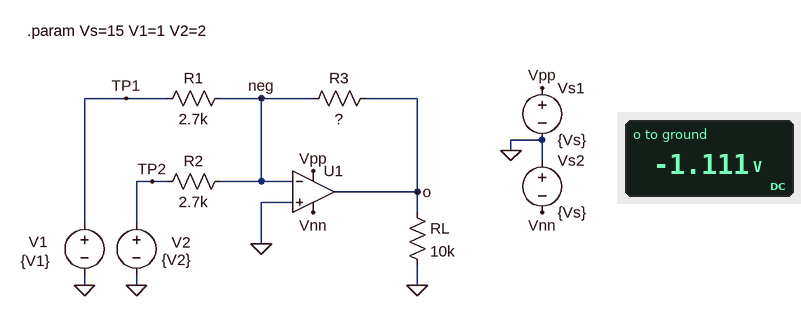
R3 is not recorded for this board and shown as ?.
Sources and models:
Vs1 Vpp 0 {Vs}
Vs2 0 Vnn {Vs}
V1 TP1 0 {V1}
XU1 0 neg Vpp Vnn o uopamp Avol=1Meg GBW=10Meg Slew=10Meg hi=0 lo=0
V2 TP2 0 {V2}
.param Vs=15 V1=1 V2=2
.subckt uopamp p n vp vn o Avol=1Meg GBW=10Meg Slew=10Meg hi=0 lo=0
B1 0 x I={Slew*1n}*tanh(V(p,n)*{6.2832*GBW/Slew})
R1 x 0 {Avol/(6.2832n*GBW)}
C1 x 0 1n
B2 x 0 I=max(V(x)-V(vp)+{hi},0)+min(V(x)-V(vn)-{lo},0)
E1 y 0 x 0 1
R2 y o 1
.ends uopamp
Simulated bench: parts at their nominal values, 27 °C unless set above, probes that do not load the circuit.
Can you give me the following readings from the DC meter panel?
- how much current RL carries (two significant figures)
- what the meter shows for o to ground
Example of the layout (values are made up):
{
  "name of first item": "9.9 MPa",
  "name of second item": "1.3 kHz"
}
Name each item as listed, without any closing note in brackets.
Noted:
{
  "how much current RL carries": "110 µA",
  "what the meter shows for o to ground": "-1.111 V"
}
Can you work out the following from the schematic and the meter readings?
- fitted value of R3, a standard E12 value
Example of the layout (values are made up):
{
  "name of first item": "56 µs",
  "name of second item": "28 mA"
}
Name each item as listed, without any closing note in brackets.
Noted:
{
  "fitted value of R3, a standard E12 value": "1 kΩ"
}
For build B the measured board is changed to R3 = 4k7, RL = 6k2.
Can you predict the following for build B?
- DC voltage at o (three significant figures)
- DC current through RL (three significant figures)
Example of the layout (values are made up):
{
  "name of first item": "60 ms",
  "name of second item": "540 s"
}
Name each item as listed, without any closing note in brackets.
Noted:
{
  "DC voltage at o": "-5.22 V",
  "DC current through RL": "842 µA"
}
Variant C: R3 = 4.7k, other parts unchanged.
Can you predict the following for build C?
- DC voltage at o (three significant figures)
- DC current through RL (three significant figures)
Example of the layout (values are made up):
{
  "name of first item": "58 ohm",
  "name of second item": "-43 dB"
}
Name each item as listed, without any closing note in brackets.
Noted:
{
  "DC voltage at o": "-5.22 V",
  "DC current through RL": "522 µA"
}
